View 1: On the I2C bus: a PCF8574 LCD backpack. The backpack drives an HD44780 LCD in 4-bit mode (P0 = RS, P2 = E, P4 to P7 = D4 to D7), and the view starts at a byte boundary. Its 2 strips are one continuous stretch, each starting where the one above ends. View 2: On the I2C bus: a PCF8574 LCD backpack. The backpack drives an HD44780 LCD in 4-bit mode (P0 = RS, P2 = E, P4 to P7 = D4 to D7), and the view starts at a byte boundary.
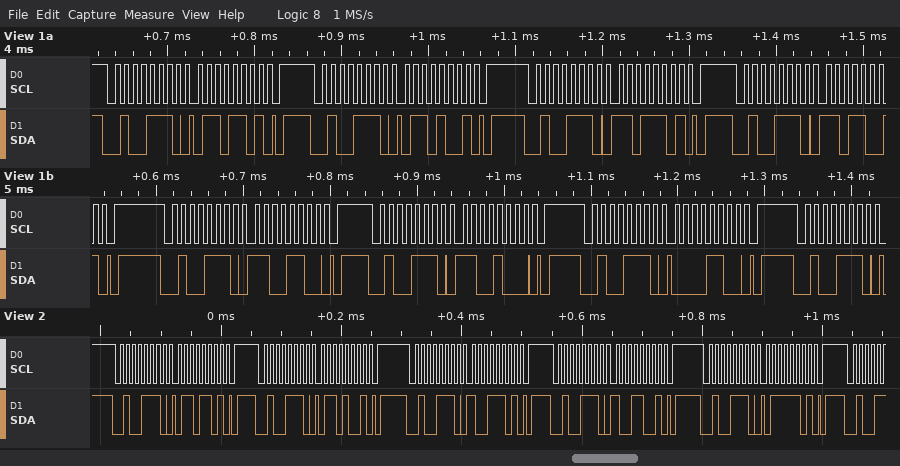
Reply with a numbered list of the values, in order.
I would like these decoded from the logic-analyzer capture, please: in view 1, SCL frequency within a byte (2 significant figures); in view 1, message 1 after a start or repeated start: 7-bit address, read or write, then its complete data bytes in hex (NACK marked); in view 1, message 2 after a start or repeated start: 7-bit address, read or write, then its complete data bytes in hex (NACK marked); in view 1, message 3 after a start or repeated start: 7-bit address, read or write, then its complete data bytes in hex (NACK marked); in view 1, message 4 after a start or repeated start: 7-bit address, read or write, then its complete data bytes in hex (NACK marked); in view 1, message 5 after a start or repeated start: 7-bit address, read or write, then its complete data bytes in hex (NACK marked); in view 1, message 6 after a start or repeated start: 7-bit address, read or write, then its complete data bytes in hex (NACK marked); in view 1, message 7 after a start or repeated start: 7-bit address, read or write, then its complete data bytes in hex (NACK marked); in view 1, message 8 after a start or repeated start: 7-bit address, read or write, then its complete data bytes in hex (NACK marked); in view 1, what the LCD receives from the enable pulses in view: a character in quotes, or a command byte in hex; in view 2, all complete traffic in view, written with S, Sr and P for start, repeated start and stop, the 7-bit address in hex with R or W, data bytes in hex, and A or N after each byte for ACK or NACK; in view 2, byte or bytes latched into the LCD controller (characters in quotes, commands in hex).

1. 100 kHz
2. 0x27 write: 6D
3. 0x27 write: 69
4. 0x27 write: DD
5. 0x27 write: D9
6. 0x27 write: CC
7. 0x27 write: C8
8. 0x27 write: 0C
9. 0x27 write
10. 'm'
11. S 27W A 6D A P S 27W A 69 A P S 27W A 9D A P S 27W A 99 A P S 27W A 7D A P
12. 'i'
